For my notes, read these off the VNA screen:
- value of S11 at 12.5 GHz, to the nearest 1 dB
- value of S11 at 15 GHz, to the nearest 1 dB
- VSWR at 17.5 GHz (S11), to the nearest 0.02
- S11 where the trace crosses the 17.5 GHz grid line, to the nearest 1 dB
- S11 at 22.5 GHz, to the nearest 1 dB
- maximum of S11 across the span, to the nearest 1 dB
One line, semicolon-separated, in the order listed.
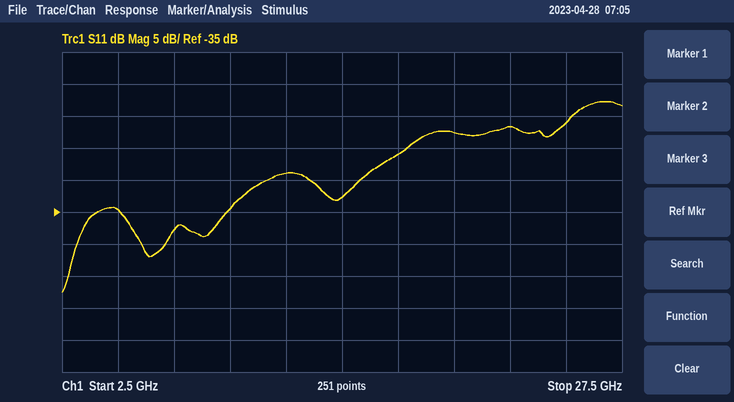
-29 dB; -33 dB; 1.10; -26 dB; -22 dB; -18 dB
